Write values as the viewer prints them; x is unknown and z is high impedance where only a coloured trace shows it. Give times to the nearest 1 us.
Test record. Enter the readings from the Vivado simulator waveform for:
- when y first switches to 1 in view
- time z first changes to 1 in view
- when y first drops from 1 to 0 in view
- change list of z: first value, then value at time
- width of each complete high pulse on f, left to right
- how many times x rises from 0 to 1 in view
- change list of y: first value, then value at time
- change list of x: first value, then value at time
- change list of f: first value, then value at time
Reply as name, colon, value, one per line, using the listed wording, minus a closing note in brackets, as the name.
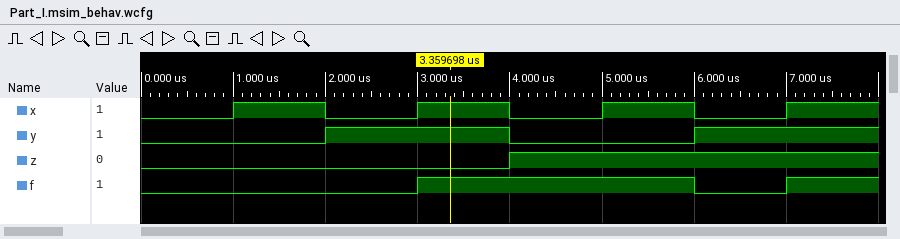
when y first switches to 1 in view: 2 us
time z first changes to 1 in view: 4 us
when y first drops from 1 to 0 in view: 4 us
change list of z: first value, then value at time: 0, 1 at 4 us
width of each complete high pulse on f, left to right: 3 us
how many times x rises from 0 to 1 in view: 4
change list of y: first value, then value at time: 0, 1 at 2 us, 0 at 4 us, 1 at 6 us
change list of x: first value, then value at time: 0, 1 at 1 us, 0 at 2 us, 1 at 3 us, 0 at 4 us, 1 at 5 us, 0 at 6 us, 1 at 7 us
change list of f: first value, then value at time: 0, 1 at 3 us, 0 at 6 us, 1 at 7 us
